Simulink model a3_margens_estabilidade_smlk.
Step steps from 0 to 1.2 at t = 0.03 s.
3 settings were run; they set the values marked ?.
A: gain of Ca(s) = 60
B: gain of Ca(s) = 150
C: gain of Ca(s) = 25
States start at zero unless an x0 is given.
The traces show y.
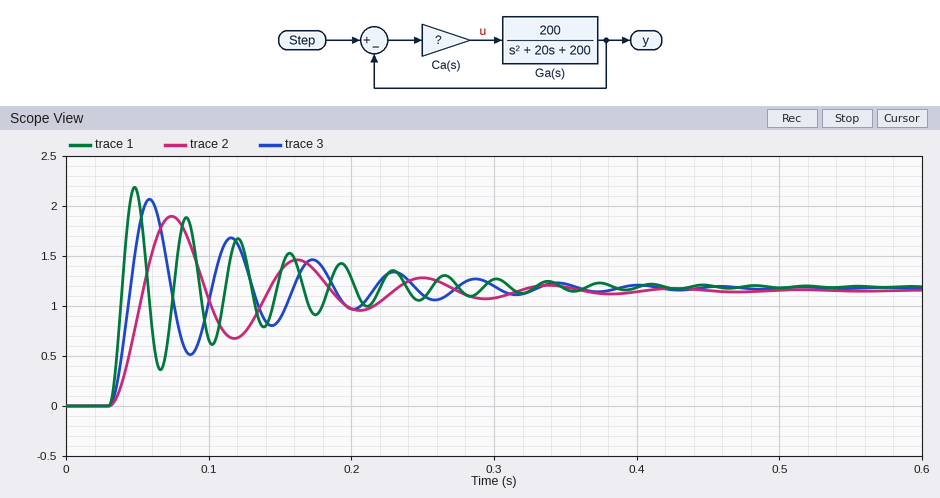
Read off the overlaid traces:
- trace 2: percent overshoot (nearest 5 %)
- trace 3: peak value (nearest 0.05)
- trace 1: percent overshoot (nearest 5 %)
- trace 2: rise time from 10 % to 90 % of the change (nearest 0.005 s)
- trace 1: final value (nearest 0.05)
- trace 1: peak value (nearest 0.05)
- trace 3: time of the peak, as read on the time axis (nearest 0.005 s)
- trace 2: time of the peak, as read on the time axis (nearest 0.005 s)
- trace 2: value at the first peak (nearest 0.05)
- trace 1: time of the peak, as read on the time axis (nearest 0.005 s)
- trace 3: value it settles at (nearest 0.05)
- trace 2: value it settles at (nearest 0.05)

65 %
2.05
85 %
0.015 s
1.20
2.20
0.060 s
0.075 s
1.90
0.050 s
1.20
1.15
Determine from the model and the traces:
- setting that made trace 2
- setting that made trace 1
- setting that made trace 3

C
B
A
